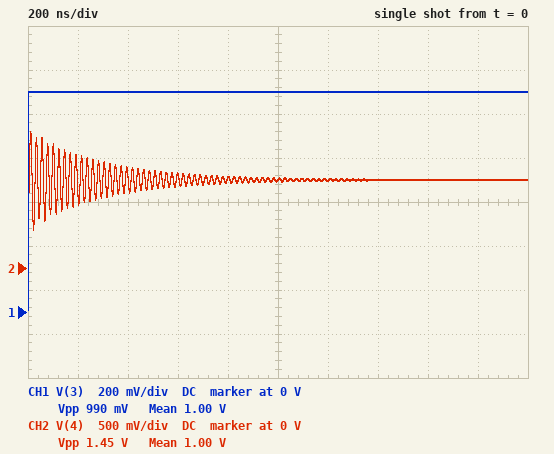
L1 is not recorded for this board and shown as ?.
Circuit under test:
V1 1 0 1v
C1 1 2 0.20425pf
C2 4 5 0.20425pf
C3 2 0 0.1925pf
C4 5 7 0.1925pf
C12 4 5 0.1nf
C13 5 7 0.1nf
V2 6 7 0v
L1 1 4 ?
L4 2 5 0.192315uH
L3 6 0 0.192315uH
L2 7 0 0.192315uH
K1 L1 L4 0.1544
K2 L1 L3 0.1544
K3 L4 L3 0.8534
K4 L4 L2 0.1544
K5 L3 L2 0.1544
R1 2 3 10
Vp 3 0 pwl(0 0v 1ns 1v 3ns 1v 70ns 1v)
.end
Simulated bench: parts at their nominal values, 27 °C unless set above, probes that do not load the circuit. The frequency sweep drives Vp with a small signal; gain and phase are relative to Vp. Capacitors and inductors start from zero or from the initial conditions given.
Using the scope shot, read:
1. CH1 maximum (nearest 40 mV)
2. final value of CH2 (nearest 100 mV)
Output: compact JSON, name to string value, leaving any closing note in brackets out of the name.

{"CH1 maximum": "1.00 V", "final value of CH2": "1.0 V"}
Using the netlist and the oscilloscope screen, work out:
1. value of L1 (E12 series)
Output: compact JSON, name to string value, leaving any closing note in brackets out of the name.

{"value of L1": "150 nH"}
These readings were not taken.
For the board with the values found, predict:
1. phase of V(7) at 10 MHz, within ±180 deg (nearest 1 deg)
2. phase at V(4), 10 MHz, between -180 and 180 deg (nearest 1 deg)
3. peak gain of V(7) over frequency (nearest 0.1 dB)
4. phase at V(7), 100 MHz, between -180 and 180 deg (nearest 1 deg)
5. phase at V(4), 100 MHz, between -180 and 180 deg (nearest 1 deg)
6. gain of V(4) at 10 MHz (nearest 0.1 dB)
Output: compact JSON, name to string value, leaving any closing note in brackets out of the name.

{"phase of V(7) at 10 MHz, within ±180 deg": "171 deg", "phase at V(4), 10 MHz, between -180 and 180 deg": "171 deg", "peak gain of V(7) over frequency": "12.4 dB", "phase at V(7), 100 MHz, between -180 and 180 deg": "4 deg", "phase at V(4), 100 MHz, between -180 and 180 deg": "4 deg", "gain of V(4) at 10 MHz": "-26.2 dB"}
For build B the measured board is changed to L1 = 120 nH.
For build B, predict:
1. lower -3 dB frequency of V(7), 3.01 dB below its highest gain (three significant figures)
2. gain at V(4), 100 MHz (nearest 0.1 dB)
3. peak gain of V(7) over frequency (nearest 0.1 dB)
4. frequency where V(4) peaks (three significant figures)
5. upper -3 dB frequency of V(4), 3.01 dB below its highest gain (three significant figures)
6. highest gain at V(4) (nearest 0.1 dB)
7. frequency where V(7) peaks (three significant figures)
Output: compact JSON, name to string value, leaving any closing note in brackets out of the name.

{"lower -3 dB frequency of V(7), 3.01 dB below its highest gain": "48.8 MHz", "gain at V(4), 100 MHz": "-5.4 dB", "peak gain of V(7) over frequency": "10.9 dB", "frequency where V(4) peaks": "50.1 MHz", "upper -3 dB frequency of V(4), 3.01 dB below its highest gain": "51.0 MHz", "highest gain at V(4)": "19.8 dB", "frequency where V(7) peaks": "49.9 MHz"}
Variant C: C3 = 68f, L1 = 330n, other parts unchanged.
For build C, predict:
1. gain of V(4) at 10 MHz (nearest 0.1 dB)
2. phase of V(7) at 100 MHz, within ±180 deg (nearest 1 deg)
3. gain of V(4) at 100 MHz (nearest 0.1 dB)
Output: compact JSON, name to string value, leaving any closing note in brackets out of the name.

{"gain of V(4) at 10 MHz": "-17.5 dB", "phase of V(7) at 100 MHz, within ±180 deg": "3 deg", "gain of V(4) at 100 MHz": "-6.5 dB"}
